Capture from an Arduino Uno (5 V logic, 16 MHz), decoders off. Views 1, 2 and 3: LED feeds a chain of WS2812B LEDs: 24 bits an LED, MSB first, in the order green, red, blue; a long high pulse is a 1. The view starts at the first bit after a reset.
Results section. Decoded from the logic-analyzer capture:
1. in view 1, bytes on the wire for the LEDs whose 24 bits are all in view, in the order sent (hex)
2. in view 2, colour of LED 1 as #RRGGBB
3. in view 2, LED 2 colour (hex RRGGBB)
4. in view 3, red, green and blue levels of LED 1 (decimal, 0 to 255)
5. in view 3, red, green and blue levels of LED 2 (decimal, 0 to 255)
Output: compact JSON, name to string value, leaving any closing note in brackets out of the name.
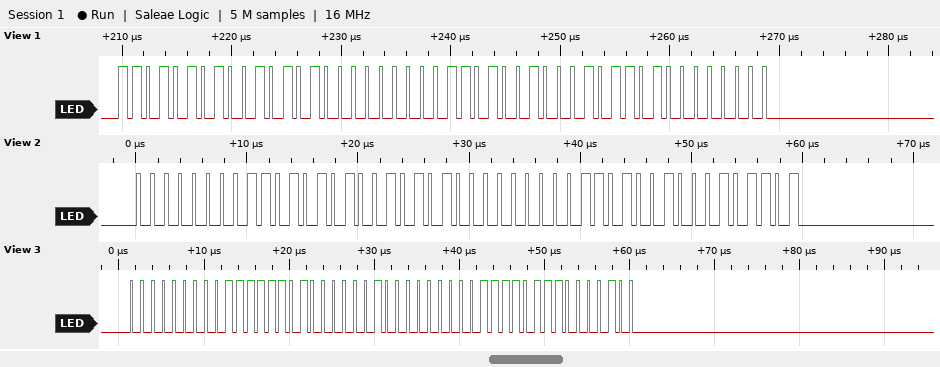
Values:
{"in view 1, bytes on the wire for the LEDs whose 24 bits are all in view, in the order sent": "D5 2A 00 D2 2D 00", "in view 2, colour of LED 1 as #RRGGBB": "#D5002A", "in view 2, LED 2 colour": "#D2002D", "in view 3, red, green and blue levels of LED 1": "126, 0, 129", "in view 3, red, green and blue levels of LED 2": "123, 0, 132"}
